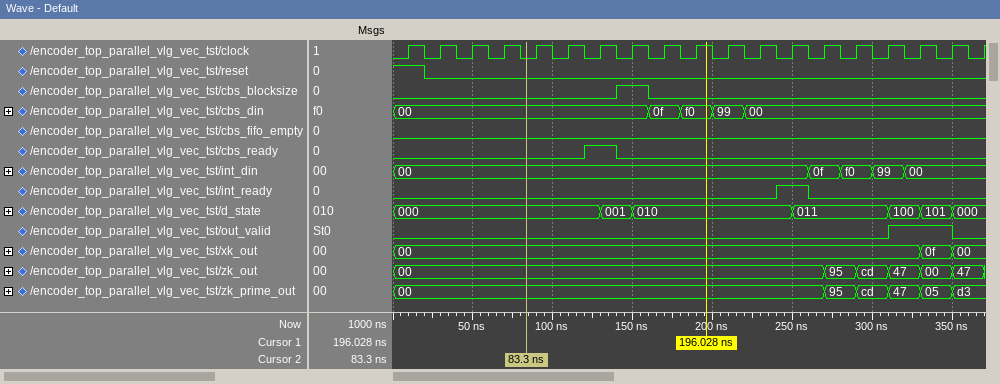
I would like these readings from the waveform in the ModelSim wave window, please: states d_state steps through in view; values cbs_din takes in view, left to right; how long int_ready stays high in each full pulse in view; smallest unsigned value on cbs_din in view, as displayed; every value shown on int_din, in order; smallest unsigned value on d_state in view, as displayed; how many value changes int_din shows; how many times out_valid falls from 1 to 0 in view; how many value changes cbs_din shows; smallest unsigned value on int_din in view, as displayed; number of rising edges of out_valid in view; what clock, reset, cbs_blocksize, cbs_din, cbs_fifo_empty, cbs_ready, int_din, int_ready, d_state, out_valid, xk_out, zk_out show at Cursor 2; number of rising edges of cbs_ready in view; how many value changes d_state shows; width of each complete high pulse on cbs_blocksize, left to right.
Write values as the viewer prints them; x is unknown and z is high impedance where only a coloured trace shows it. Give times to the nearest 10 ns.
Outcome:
000, 001, 010, 011, 100, 101, 000
00, 0f, f0, 99, 00
20 ns
00
00, 0f, f0, 99, 00
000
4
1
4
00
1
clock=0, reset=0, cbs_blocksize=0, cbs_din=00, cbs_fifo_empty=0, cbs_ready=0, int_din=00, int_ready=0, d_state=000, out_valid=0, xk_out=00, zk_out=00
1
6
20 ns
